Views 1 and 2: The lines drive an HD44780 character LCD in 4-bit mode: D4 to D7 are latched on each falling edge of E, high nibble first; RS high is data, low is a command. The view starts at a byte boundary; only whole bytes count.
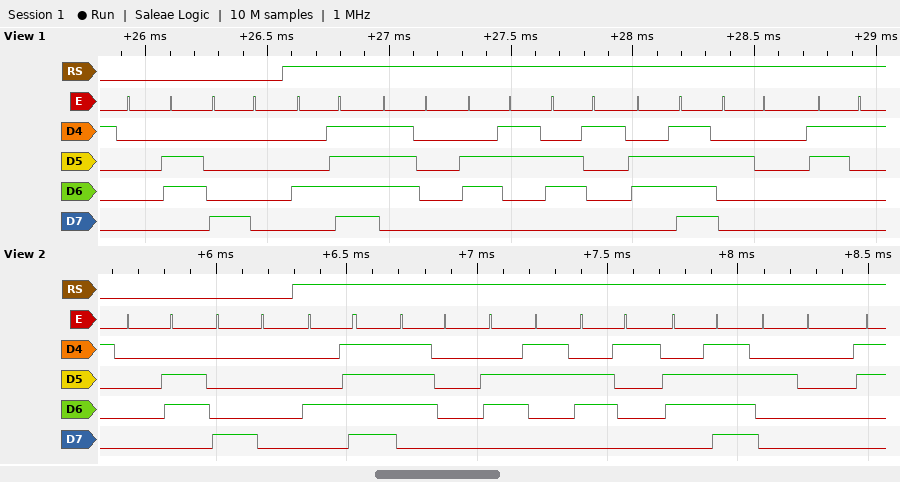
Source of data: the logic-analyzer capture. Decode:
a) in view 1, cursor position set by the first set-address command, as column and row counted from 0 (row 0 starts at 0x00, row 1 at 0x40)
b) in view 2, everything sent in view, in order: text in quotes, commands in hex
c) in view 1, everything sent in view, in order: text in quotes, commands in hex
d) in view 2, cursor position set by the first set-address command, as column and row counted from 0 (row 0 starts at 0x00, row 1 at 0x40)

column 0, row 0
0x06 0x80 "Opcao "
0x06 0x80 "Opcao 1"
column 0, row 0
